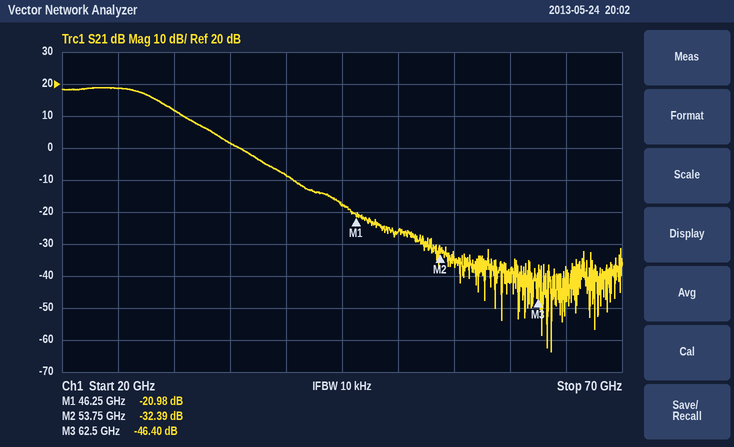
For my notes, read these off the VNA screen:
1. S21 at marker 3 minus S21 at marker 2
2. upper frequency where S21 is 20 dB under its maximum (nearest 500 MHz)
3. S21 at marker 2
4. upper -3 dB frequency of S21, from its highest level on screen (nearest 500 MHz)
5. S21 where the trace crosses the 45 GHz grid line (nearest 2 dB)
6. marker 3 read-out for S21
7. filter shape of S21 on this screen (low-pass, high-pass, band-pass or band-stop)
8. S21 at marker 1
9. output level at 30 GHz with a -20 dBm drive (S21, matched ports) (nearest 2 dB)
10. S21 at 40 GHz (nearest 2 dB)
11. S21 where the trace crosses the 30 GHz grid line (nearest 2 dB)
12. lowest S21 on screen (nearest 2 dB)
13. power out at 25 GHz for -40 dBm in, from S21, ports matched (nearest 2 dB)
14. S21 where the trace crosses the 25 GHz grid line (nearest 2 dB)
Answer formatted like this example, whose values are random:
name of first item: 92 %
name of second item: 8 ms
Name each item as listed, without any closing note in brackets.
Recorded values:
S21 at marker 3 minus S21 at marker 2: -14.01 dB
upper frequency where S21 is 20 dB under its maximum: 36.5 GHz
S21 at marker 2: -32.39 dB
upper -3 dB frequency of S21, from its highest level on screen: 28.0 GHz
S21 where the trace crosses the 45 GHz grid line: -18 dB
marker 3 read-out for S21: -46.40 dB
filter shape of S21 on this screen: low-pass
S21 at marker 1: -20.98 dB
output level at 30 GHz with a -20 dBm drive (S21, matched ports): -8 dBm
S21 at 40 GHz: -8 dB
S21 where the trace crosses the 30 GHz grid line: 12 dB
lowest S21 on screen: -64 dB
power out at 25 GHz for -40 dBm in, from S21, ports matched: -22 dBm
S21 where the trace crosses the 25 GHz grid line: 18 dB
